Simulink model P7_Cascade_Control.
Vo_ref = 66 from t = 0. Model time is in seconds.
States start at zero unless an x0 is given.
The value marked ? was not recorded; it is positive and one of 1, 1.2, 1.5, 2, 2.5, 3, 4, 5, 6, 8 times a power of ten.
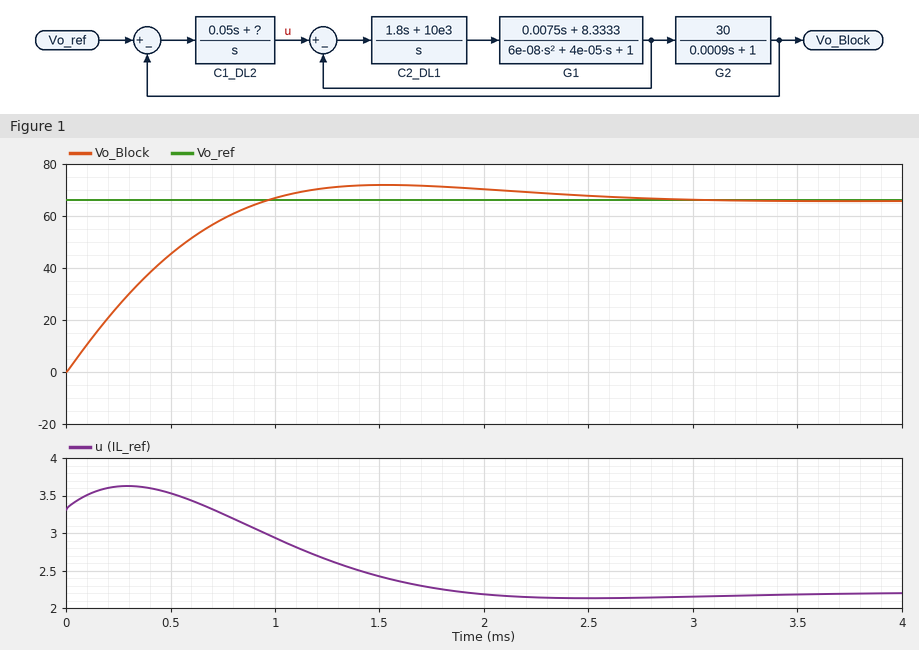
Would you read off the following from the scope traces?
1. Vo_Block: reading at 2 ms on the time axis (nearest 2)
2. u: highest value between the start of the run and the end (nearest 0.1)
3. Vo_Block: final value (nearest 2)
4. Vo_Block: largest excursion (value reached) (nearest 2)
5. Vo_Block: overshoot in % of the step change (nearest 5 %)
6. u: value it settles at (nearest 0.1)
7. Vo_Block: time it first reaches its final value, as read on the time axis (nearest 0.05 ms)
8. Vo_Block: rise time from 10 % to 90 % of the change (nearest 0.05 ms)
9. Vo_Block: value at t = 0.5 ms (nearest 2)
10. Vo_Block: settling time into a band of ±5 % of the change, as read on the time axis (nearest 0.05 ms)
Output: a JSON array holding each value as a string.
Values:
["70", "3.6", "66", "72", "10 %", "2.2", "0.95 ms", "0.70 ms", "46", "2.20 ms"]
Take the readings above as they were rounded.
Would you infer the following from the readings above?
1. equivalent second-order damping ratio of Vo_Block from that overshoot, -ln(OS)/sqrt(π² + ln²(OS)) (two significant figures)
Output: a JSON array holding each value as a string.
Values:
["0.59"]
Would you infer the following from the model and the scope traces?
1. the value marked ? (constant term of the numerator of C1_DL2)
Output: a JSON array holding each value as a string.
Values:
["120"]
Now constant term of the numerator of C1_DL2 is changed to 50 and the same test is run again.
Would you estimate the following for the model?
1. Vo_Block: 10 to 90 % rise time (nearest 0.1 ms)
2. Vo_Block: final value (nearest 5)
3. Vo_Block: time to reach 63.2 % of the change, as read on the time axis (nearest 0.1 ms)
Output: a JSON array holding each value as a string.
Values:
["1.5 ms", "65", "0.6 ms"]
